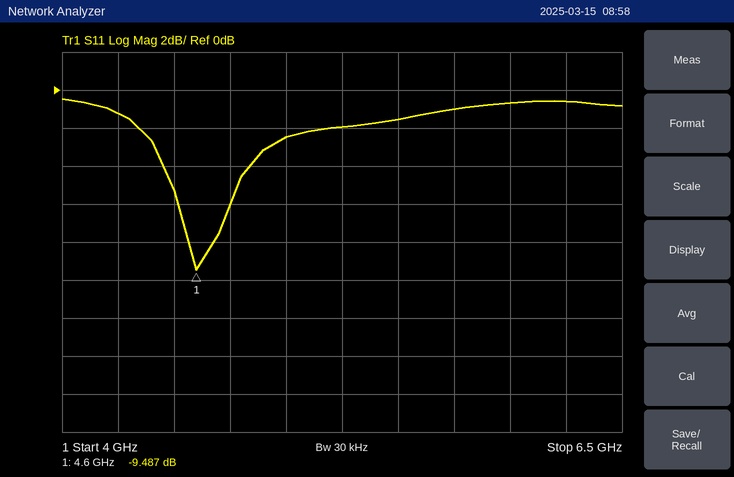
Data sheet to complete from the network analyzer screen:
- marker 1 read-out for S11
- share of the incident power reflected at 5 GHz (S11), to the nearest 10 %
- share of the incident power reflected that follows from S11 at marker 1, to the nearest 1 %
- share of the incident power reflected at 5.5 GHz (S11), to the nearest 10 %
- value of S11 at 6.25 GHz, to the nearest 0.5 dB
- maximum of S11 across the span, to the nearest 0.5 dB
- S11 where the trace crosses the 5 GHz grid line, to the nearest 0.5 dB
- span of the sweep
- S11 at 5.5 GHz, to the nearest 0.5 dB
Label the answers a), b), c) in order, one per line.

a) -9.487 dB
b) 60 %
c) 11 %
d) 70 %
e) -0.5 dB
f) -0.5 dB
g) -2.5 dB
h) 2.5 GHz
i) -1.5 dB
